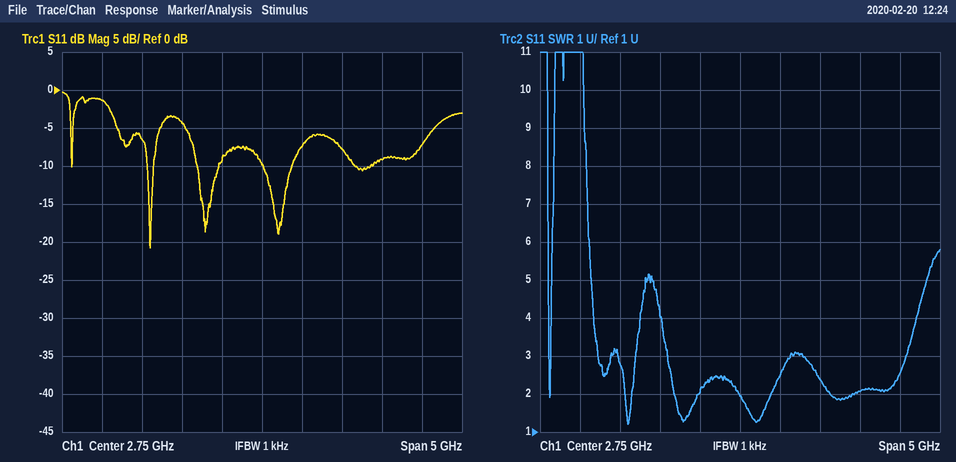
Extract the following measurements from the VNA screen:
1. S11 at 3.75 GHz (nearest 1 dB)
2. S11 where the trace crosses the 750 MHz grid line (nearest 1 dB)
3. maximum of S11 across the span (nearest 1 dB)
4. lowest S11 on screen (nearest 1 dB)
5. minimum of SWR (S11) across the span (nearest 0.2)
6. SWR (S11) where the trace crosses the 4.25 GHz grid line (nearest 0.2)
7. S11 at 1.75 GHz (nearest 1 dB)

-8 dB
-1 dB
0 dB
-21 dB
1.2
2.0
-4 dB
